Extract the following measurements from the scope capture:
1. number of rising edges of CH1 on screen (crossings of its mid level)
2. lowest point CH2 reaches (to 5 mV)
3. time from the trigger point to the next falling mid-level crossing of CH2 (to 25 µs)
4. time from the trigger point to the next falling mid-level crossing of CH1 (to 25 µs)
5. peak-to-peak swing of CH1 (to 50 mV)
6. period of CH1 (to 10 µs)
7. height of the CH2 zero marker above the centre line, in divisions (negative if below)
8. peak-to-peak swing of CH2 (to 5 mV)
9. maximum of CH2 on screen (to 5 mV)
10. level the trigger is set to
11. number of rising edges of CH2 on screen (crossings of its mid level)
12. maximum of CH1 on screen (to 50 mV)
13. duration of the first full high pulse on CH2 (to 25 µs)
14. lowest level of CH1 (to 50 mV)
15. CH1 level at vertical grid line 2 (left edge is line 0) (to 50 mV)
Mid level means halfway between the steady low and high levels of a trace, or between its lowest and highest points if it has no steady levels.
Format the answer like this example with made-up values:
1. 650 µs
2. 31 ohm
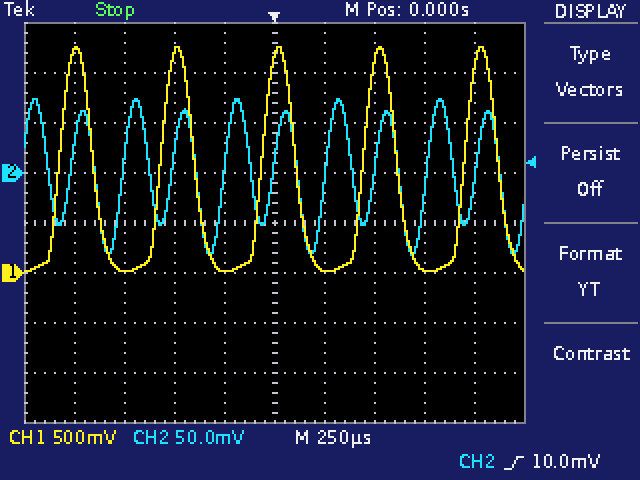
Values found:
1. 5
2. -80 mV
3. 125 µs
4. 100 µs
5. 2.25 V
6. 510 µs
7. +1.0 div
8. 155 mV
9. 75 mV
10. 10.0 mV
11. 9
12. 2.25 V
13. 125 µs
14. 0 mV
15. 0 mV
